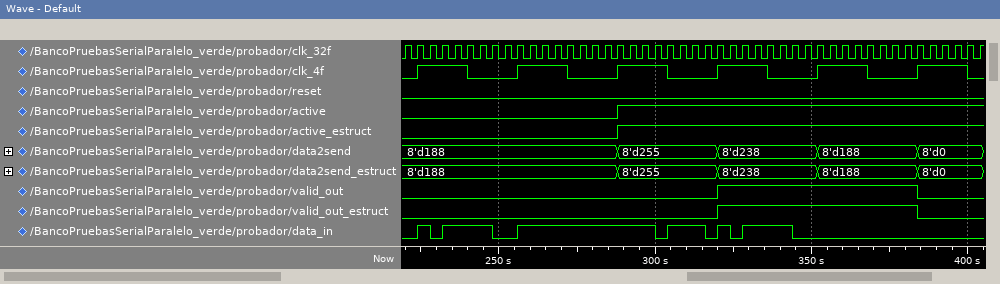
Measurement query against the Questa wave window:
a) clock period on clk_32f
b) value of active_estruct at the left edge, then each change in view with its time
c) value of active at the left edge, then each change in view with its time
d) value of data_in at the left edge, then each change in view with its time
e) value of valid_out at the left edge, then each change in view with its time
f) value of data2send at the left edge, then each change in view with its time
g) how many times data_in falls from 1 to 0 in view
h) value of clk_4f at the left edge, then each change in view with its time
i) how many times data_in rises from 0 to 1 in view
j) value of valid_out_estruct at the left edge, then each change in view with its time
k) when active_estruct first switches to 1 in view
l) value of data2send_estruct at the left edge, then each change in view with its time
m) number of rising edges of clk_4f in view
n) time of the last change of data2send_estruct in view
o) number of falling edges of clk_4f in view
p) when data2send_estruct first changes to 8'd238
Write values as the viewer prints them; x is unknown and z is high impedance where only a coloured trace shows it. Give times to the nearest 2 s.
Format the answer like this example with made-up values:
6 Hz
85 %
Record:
4 s
0, 1 at 288 s
0, 1 at 288 s
0, 1 at 224 s, 0 at 228 s, 1 at 232 s, 0 at 248 s, 1 at 256 s, 0 at 300 s, 1 at 304 s, 0 at 316 s, 1 at 320 s, 0 at 324 s, 1 at 328 s, 0 at 344 s
0, 1 at 320 s, 0 at 384 s
8'd188, 8'd255 at 288 s, 8'd238 at 320 s, 8'd188 at 352 s, 8'd0 at 384 s
6
0, 1 at 224 s, 0 at 240 s, 1 at 256 s, 0 at 272 s, 1 at 288 s, 0 at 304 s, 1 at 320 s, 0 at 336 s, 1 at 352 s, 0 at 368 s, 1 at 384 s, 0 at 400 s
6
0, 1 at 320 s, 0 at 384 s
288 s
8'd188, 8'd255 at 288 s, 8'd238 at 320 s, 8'd188 at 352 s, 8'd0 at 384 s
6
384 s
6
320 s
